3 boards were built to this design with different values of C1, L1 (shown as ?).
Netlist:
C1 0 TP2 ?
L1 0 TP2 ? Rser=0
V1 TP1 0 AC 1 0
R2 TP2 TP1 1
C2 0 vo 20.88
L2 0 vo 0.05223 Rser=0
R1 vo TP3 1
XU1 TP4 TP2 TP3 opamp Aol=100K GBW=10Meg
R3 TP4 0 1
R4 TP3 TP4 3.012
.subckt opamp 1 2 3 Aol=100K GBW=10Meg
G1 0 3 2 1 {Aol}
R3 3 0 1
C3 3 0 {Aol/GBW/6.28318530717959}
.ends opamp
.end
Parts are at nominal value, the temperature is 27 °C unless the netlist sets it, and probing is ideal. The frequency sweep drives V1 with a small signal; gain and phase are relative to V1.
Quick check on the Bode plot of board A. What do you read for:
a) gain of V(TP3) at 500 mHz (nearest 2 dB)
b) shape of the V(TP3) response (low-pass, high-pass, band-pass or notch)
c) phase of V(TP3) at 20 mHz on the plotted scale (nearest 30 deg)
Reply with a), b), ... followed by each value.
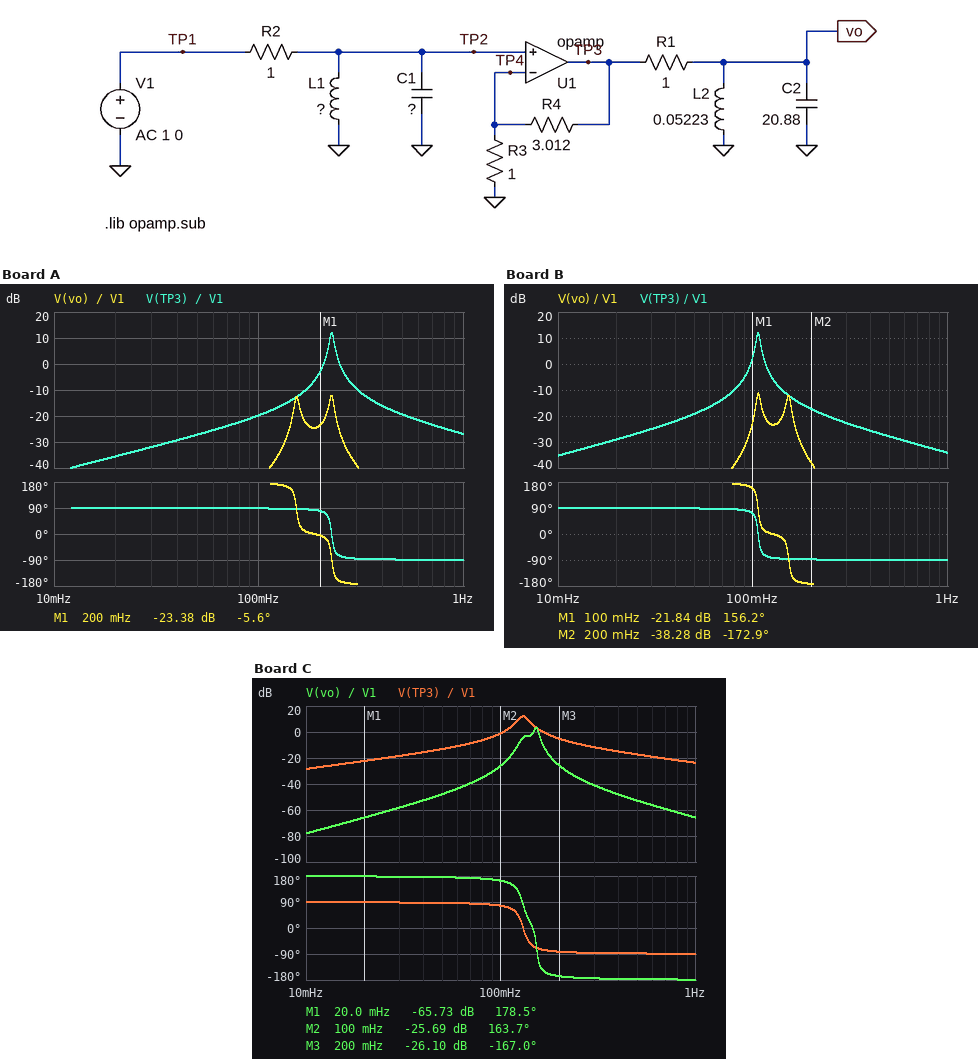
a) -20 dB
b) band-pass
c) 90 deg
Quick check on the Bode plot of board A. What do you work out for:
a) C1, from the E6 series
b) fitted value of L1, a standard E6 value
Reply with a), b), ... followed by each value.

a) 15 F
b) 33 mH
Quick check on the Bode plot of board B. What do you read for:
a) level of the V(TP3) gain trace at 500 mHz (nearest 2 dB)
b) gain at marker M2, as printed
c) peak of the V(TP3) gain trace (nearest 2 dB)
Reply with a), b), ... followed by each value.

a) -28 dB
b) -38.28 dB
c) 12 dB
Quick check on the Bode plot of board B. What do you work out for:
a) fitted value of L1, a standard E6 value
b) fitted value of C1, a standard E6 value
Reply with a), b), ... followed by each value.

a) 68 mH
b) 33 F
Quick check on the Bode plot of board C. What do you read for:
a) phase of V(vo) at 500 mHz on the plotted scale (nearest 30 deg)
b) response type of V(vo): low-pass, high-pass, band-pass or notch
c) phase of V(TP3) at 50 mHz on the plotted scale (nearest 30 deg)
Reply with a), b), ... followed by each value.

a) -180 deg
b) band-pass
c) 90 deg
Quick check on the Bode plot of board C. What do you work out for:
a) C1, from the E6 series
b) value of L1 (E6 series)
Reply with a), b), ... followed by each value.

a) 10 F
b) 150 mH
